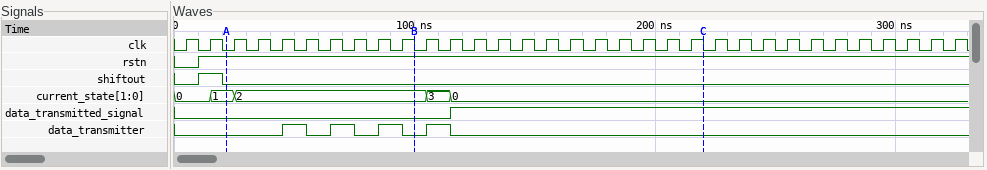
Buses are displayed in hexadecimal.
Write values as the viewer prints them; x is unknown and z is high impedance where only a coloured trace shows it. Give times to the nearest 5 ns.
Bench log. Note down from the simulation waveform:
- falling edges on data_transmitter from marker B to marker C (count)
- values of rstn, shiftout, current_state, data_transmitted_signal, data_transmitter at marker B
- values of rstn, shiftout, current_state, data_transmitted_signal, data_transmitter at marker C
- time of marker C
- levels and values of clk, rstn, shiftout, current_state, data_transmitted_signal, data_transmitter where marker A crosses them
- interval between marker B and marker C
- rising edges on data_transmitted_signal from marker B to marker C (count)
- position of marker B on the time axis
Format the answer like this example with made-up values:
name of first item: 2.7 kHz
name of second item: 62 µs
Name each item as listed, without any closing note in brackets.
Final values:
falling edges on data_transmitter from marker B to marker C: 1
values of rstn, shiftout, current_state, data_transmitted_signal, data_transmitter at marker B: rstn=1, shiftout=0, current_state=2, data_transmitted_signal=0, data_transmitter=0
values of rstn, shiftout, current_state, data_transmitted_signal, data_transmitter at marker C: rstn=1, shiftout=0, current_state=0, data_transmitted_signal=1, data_transmitter=0
time of marker C: 220 ns
levels and values of clk, rstn, shiftout, current_state, data_transmitted_signal, data_transmitter where marker A crosses them: clk=0, rstn=1, shiftout=0, current_state=1, data_transmitted_signal=0, data_transmitter=0
interval between marker B and marker C: 120 ns
rising edges on data_transmitted_signal from marker B to marker C: 1
position of marker B on the time axis: 100 ns
